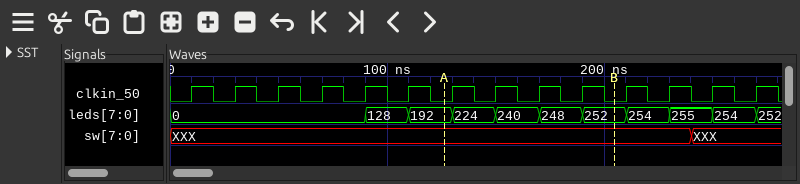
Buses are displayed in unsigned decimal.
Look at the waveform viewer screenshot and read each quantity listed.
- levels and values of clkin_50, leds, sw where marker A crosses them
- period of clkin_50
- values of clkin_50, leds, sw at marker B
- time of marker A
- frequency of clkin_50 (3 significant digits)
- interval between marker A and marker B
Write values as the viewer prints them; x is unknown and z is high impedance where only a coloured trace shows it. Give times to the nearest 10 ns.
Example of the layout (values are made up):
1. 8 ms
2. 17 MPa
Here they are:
1. clkin_50=0, leds=192, sw=XXX
2. 20 ns
3. clkin_50=0, leds=252, sw=XXX
4. 130 ns
5. 50.0 MHz
6. 80 ns
